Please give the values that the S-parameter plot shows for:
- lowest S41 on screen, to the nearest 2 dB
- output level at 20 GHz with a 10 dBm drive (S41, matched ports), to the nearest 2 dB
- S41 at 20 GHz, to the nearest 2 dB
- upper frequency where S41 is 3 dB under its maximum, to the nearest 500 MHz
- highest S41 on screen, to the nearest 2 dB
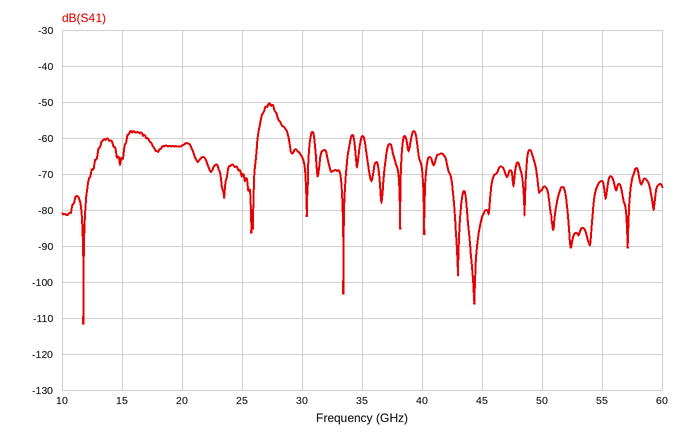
-112 dB
-52 dBm
-62 dB
28.0 GHz
-50 dB
